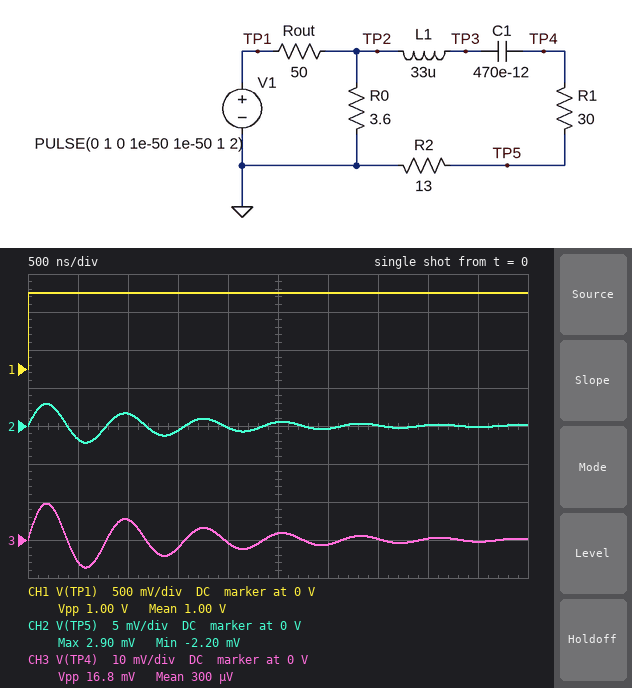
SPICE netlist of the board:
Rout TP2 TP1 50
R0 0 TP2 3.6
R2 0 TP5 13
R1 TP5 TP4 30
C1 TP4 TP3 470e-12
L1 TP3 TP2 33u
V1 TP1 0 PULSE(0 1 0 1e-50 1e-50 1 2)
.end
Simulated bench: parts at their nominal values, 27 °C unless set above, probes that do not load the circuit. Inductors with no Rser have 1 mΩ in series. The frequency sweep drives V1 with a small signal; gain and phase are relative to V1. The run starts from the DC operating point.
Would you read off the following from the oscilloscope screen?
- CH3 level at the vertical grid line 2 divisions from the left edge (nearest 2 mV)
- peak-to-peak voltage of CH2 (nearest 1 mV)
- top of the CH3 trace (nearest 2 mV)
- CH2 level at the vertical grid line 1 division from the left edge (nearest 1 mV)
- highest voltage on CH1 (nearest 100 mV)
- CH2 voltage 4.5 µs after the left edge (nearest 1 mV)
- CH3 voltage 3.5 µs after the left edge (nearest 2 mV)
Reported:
6 mV
5 mV
10 mV
-2 mV
1.0 V
0 V
0 V
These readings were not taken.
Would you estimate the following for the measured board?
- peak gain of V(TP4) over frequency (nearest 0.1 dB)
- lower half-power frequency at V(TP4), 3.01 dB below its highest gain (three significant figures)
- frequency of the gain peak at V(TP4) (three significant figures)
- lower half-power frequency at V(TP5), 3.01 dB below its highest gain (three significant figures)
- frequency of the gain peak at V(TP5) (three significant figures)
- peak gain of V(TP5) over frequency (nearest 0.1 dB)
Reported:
-24.1 dB
1.17 MHz
1.28 MHz
1.17 MHz
1.28 MHz
-34.5 dB
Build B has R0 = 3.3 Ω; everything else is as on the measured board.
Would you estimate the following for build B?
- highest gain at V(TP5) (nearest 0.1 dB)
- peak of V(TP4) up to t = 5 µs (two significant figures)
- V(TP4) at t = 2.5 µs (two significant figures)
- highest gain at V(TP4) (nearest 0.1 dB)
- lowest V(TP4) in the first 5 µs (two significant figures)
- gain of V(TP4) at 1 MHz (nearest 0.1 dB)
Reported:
-35.2 dB
8.8 mV
1.6 mV
-24.8 dB
-6.7 mV
-34.4 dB
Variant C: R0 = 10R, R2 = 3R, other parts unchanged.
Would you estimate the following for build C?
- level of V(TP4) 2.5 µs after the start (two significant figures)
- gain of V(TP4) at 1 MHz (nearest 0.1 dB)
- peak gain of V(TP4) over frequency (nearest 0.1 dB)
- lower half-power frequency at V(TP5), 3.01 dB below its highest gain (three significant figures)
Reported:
4.0 mV
-28.0 dB
-17.5 dB
1.18 MHz
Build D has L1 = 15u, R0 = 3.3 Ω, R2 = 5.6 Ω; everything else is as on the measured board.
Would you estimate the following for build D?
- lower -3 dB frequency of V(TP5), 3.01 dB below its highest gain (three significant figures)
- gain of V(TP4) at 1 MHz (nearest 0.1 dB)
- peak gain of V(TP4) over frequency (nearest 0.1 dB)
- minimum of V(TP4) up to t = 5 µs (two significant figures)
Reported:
1.70 MHz
-41.0 dB
-24.9 dB
-7.5 mV
